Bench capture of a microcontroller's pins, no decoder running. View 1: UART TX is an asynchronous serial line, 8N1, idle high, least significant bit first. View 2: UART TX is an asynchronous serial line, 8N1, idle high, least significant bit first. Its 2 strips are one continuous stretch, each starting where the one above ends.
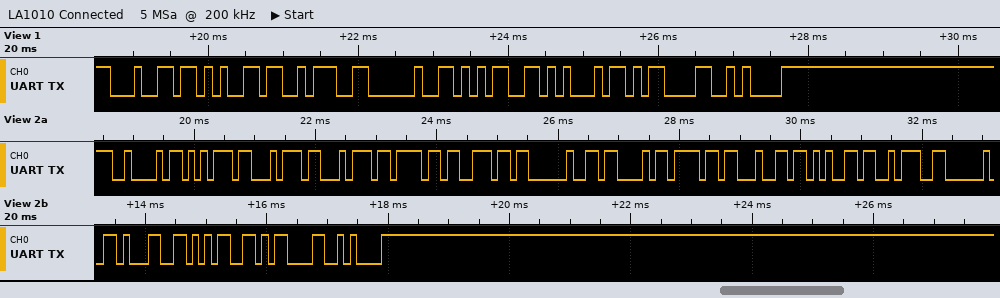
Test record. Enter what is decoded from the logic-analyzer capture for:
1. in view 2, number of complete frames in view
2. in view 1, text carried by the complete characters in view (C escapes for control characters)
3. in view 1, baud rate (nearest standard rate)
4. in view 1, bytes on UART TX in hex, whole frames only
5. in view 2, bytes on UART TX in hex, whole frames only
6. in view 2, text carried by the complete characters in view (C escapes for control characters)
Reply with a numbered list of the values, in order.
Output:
1. 17
2. "de: 5E\r\n"
3. 9600 baud
4. 64 65 3A 20 35 45 0D 0A
5. 42 75 74 74 6F 6E 20 43 6F 64 65 3A 20 31 35 0D 0A
6. "Button Code: 15\r\n"
